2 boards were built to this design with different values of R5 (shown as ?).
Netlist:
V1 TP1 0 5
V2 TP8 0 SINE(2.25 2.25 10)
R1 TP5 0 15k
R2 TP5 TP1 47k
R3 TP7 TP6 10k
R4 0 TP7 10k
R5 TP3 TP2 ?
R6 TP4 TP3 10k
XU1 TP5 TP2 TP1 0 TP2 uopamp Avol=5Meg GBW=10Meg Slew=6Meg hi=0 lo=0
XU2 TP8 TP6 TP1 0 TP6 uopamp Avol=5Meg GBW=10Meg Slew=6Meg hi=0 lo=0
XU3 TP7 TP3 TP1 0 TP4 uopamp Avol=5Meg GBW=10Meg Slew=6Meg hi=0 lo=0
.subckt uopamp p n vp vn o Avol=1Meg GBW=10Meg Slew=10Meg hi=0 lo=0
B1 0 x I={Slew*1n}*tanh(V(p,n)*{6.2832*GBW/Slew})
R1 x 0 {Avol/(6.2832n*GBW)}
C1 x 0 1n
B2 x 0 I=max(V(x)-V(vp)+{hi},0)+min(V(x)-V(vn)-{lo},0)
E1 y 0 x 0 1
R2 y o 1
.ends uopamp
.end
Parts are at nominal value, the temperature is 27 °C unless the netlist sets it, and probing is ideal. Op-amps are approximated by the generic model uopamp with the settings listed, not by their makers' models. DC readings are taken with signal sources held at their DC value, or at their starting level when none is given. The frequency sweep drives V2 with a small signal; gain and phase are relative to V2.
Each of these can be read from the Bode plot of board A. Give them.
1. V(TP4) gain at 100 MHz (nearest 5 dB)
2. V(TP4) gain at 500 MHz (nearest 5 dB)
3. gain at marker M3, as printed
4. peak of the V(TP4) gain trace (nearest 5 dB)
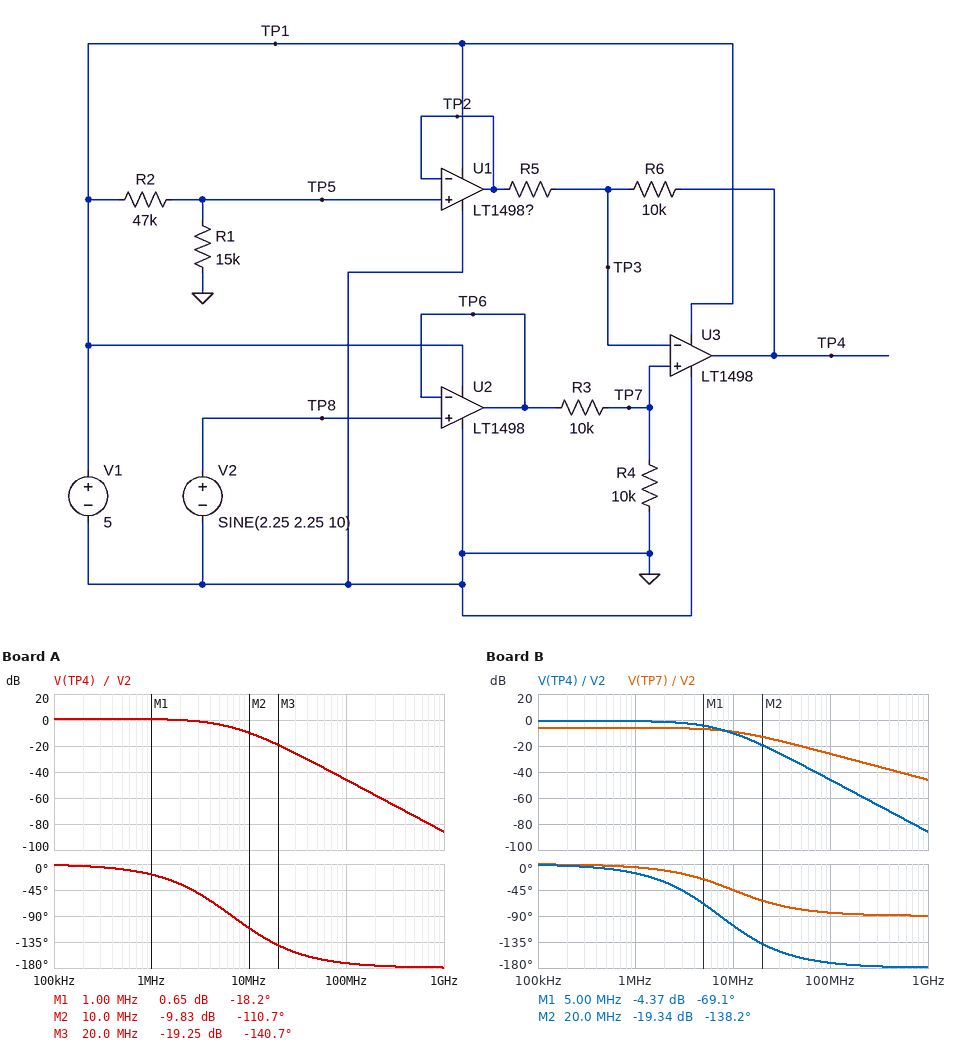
-45 dB
-75 dB
-19.25 dB
0 dB
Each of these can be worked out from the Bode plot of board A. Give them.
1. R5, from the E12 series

8.2 kΩ
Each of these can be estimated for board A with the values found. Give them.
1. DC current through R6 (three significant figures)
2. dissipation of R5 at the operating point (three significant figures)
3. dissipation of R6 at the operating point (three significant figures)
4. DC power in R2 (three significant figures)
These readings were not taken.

10.3 µA
874 nW
1.07 µW
306 µW
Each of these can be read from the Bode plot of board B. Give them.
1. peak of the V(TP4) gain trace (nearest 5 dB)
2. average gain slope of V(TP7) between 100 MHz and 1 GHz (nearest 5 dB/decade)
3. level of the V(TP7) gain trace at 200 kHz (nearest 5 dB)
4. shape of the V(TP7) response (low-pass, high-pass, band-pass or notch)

0 dB
-20 dB/decade
-5 dB
low-pass
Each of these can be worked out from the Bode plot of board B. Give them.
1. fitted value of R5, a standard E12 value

12 kΩ
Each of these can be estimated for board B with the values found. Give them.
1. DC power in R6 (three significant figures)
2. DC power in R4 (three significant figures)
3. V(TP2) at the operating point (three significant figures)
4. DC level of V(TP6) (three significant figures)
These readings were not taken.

498 nW
127 µW
1.21 V
2.25 V
